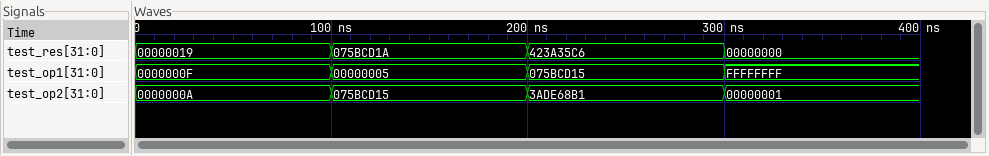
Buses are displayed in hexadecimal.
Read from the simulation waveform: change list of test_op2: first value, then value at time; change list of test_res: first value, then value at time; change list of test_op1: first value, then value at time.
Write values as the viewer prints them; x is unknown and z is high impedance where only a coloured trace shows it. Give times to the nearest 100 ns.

0000000A, 075BCD15 at 100 ns, 3ADE68B1 at 200 ns, 00000001 at 300 ns
00000019, 075BCD1A at 100 ns, 423A35C6 at 200 ns, 00000000 at 300 ns
0000000F, 00000005 at 100 ns, 075BCD15 at 200 ns, FFFFFFFF at 300 ns
